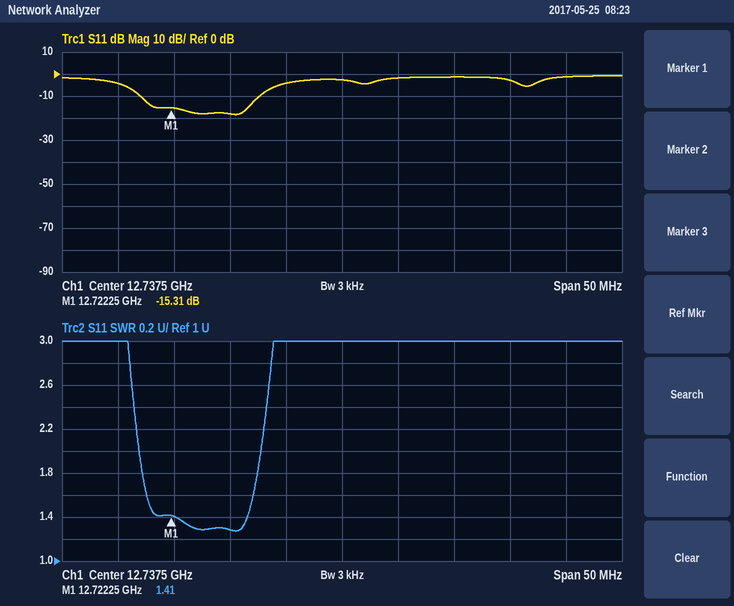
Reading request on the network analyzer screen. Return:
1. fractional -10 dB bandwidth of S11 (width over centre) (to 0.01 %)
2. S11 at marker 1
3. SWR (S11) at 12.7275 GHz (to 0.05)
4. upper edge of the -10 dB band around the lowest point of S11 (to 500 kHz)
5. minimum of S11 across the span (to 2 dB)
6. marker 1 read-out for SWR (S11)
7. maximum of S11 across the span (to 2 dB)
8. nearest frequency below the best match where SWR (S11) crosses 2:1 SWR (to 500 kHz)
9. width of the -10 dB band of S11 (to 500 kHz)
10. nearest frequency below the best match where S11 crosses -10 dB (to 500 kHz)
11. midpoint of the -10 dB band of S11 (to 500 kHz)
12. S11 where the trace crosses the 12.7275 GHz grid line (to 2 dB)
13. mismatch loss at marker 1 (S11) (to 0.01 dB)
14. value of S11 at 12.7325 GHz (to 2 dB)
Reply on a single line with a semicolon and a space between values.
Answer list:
0.08 %; -15.31 dB; 1.30; 12.7300 GHz; -18 dB; 1.41; 0 dB; 12.7195 GHz; 10.5 MHz; 12.7195 GHz; 12.7250 GHz; -18 dB; 0.13 dB; -4 dB
